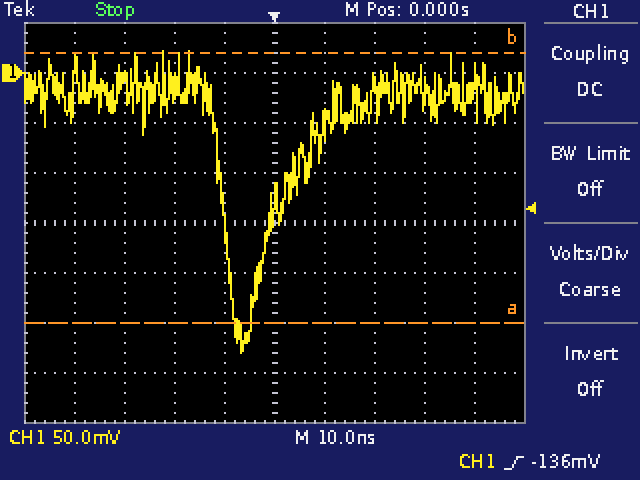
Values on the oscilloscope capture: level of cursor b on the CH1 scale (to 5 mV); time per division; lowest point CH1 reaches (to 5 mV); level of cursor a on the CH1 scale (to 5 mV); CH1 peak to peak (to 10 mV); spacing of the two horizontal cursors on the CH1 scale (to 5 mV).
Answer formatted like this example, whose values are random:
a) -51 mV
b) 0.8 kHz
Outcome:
a) 20 mV
b) 10 ns
c) -280 mV
d) -250 mV
e) 300 mV
f) 270 mV
